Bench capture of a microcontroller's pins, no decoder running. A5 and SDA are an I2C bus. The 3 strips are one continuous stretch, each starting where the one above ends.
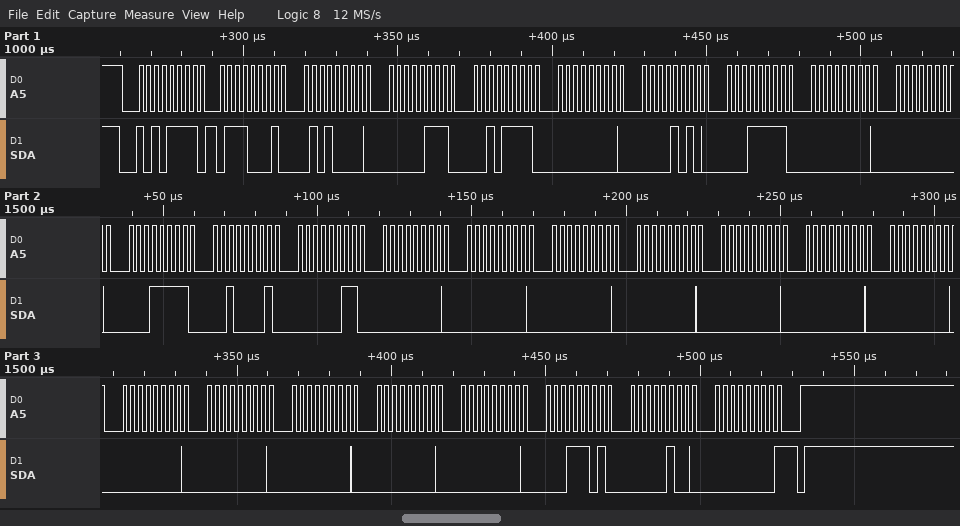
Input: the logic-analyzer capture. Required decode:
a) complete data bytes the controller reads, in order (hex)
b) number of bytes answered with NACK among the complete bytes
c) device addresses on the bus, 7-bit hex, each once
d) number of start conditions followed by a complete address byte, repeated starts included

71 50 07 2F 00 0A 1F 00 00 1F 21 03 00 00 00 00 00 00 00 00 00 00 00 00 1D 04 00
1
0x57
1
